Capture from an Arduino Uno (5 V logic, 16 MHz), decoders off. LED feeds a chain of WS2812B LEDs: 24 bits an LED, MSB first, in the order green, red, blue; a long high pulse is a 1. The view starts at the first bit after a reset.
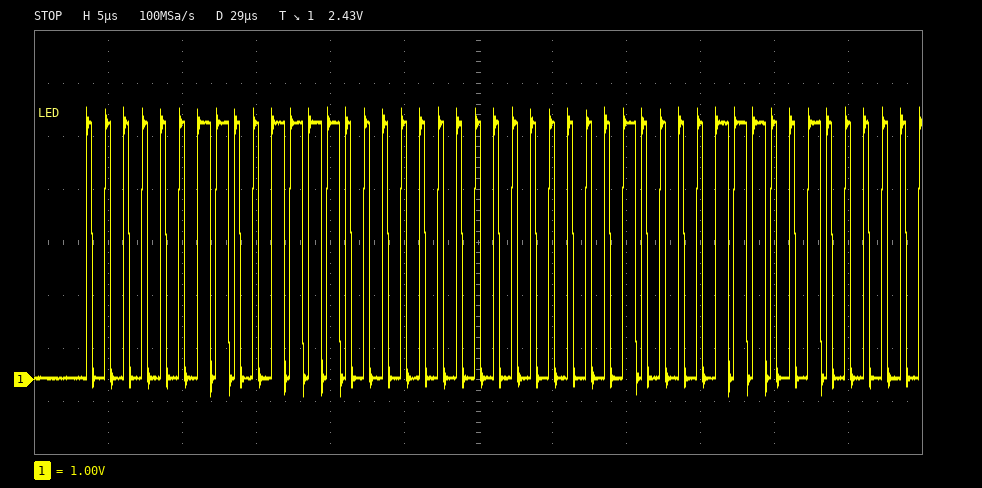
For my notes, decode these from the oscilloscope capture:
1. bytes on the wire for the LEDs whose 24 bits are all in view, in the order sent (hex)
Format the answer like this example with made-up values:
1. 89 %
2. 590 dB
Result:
1. 03 3C 00
